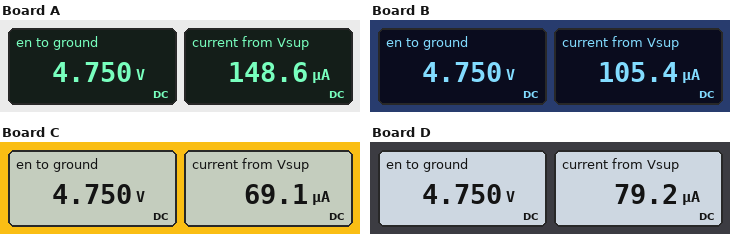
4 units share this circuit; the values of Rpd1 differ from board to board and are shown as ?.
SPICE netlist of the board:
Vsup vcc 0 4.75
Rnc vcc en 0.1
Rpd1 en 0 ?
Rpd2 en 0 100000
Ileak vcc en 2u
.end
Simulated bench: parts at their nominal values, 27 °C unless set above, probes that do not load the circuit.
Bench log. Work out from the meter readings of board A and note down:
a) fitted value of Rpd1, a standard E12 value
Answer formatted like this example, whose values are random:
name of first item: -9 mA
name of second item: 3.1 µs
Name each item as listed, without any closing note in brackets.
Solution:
fitted value of Rpd1, a standard E12 value: 47 kΩ
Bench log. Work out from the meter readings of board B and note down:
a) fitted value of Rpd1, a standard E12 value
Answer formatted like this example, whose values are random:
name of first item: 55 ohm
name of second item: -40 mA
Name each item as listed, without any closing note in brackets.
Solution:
fitted value of Rpd1, a standard E12 value: 82 kΩ
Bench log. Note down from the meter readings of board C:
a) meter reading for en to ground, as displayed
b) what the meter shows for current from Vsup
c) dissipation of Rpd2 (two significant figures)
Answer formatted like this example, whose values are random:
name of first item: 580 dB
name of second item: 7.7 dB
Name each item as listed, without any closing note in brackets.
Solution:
meter reading for en to ground, as displayed: 4.750 V
what the meter shows for current from Vsup: 69.1 µA
dissipation of Rpd2: 230 µW
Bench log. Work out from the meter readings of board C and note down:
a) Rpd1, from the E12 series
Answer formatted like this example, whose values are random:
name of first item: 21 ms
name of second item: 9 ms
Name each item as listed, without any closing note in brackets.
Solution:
Rpd1, from the E12 series: 220 kΩ
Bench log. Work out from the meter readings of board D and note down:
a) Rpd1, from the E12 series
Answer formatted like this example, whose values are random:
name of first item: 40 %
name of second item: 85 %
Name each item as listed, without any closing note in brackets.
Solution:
Rpd1, from the E12 series: 150 kΩ
